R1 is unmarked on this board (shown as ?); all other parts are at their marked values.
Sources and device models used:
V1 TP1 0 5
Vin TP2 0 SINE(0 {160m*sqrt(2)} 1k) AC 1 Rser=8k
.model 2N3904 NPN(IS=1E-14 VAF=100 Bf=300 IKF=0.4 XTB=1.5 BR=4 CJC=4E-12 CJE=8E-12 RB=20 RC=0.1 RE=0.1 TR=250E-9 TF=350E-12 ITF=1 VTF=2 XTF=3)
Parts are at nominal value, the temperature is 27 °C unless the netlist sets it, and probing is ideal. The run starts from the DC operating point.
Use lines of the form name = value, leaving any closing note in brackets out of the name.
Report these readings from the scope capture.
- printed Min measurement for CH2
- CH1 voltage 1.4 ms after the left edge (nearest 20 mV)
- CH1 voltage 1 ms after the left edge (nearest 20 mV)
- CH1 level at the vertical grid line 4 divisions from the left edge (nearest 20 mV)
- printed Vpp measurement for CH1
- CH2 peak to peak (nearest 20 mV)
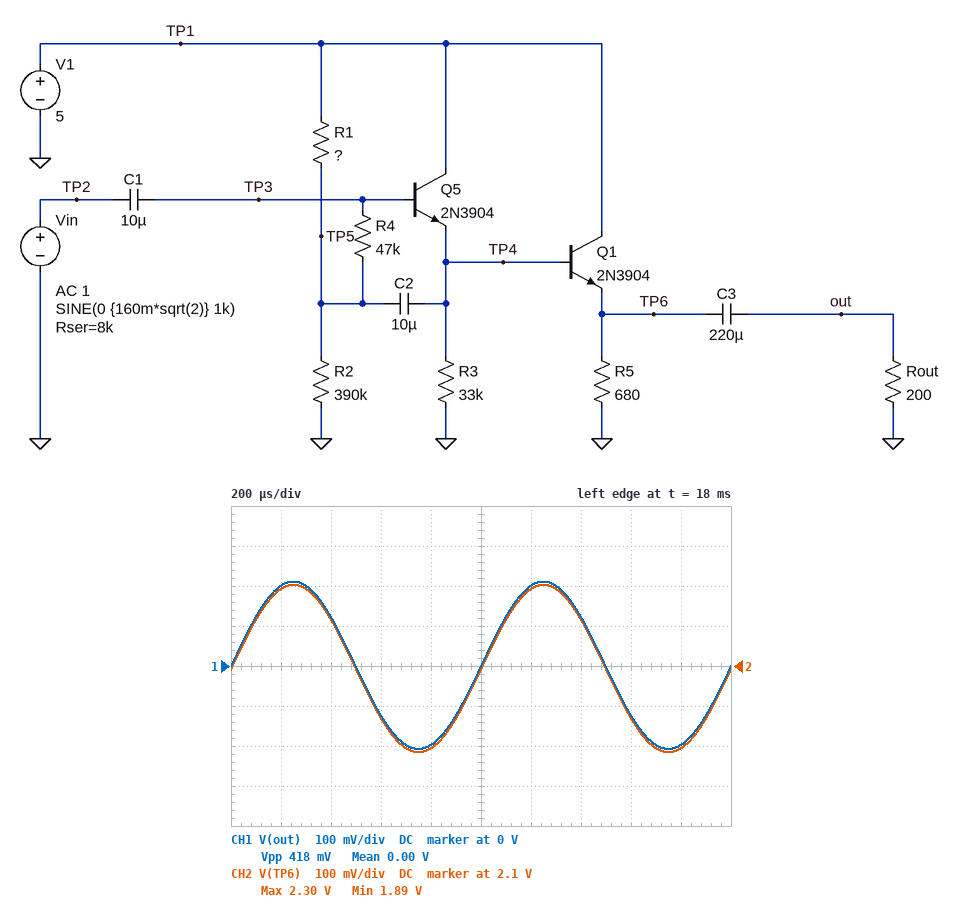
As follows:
printed Min measurement for CH2 = 1.89 V
CH1 voltage 1.4 ms after the left edge = 120 mV
CH1 voltage 1 ms after the left edge = 0 V
CH1 level at the vertical grid line 4 divisions from the left edge = -200 mV
printed Vpp measurement for CH1 = 418 mV
CH2 peak to peak = 420 mV
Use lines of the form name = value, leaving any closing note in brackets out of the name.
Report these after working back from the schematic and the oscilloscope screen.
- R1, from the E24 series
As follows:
R1, from the E24 series = 180 kΩ
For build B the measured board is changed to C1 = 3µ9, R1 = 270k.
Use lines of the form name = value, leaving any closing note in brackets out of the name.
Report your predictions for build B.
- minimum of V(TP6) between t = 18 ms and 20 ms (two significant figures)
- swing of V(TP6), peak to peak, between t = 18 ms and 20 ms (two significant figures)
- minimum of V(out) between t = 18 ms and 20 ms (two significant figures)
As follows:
minimum of V(TP6) between t = 18 ms and 20 ms = 1.4 V
swing of V(TP6), peak to peak, between t = 18 ms and 20 ms = 410 mV
minimum of V(out) between t = 18 ms and 20 ms = -200 mV
